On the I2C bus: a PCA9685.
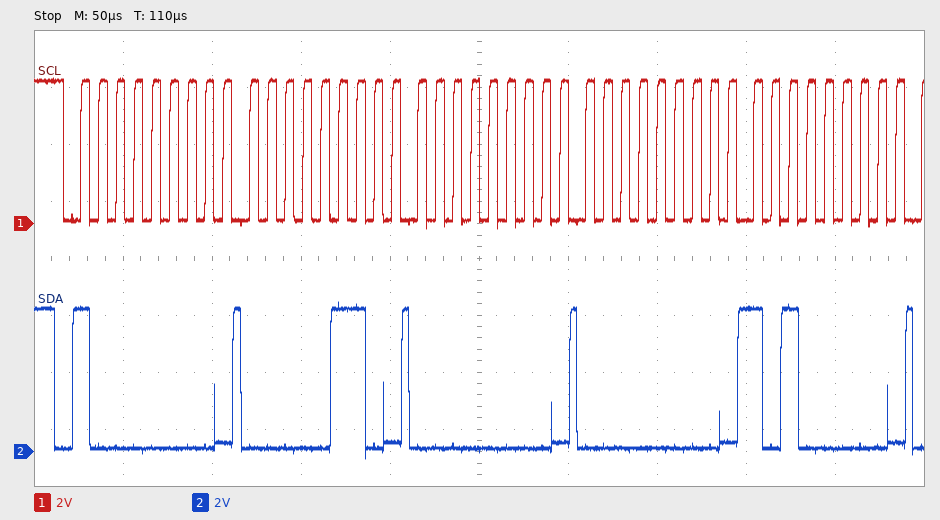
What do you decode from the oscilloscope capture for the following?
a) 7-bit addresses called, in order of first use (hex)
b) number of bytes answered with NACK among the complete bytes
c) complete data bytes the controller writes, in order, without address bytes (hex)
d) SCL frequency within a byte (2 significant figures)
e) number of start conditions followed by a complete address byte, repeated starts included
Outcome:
0x40
0
06 00 00 A0
100 kHz
1
